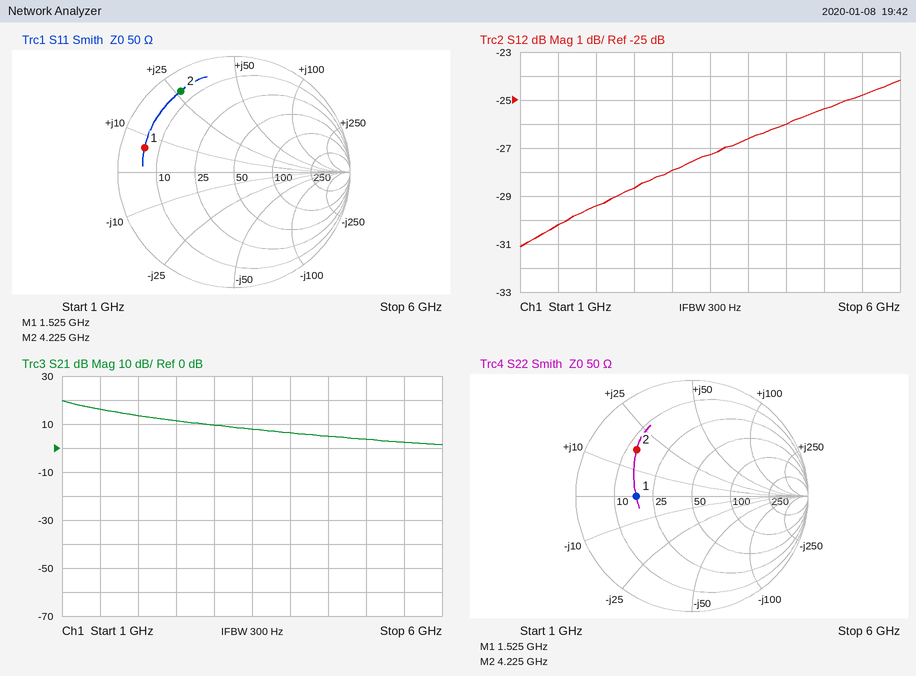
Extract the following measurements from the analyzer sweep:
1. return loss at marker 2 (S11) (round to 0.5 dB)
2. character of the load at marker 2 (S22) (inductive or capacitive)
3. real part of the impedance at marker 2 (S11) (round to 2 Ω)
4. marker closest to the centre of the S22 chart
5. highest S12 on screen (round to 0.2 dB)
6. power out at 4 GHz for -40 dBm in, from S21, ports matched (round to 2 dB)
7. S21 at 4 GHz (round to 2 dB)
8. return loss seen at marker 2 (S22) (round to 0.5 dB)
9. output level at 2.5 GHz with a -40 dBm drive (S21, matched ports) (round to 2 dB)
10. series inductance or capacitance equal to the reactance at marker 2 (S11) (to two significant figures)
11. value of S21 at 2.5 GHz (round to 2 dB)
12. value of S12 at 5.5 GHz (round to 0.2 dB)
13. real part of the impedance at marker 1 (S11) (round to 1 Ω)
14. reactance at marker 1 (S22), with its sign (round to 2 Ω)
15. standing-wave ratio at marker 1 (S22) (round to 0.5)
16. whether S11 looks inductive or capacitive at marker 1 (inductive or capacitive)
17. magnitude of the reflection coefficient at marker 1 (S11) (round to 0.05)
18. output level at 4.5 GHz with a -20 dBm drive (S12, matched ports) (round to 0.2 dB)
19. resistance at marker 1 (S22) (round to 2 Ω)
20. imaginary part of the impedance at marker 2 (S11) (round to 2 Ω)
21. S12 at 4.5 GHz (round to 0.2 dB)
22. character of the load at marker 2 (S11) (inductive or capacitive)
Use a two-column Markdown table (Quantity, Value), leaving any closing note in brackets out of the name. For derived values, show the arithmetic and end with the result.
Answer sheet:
| Quantity | Value |
|---|---|
| return loss at marker 2 (S11) | 1.5 dB |
| character of the load at marker 2 (S22) | inductive |
| real part of the impedance at marker 2 (S11) | 6 Ω |
| marker closest to the centre of the S22 chart | marker 1 |
| highest S12 on screen | -24.2 dB |
| power out at 4 GHz for -40 dBm in, from S21, ports matched | -40 dBm + (6 dB) = -34 dBm |
| S21 at 4 GHz | 6 dB |
| return loss seen at marker 2 (S22) | 4.0 dB |
| output level at 2.5 GHz with a -40 dBm drive (S21, matched ports) | -40 dBm + (12 dB) = -28 dBm |
| series inductance or capacitance equal to the reactance at marker 2 (S11) | L = 26 Ω/(2π × 4.225 GHz) ≈ 1.0 nH |
| value of S21 at 2.5 GHz | 12 dB |
| value of S12 at 5.5 GHz | -24.8 dB |
| real part of the impedance at marker 1 (S11) | 6 Ω |
| reactance at marker 1 (S22), with its sign | 0 Ω |
| standing-wave ratio at marker 1 (S22) | 3.0 |
| whether S11 looks inductive or capacitive at marker 1 | inductive |
| magnitude of the reflection coefficient at marker 1 (S11) | 0.80 |
| output level at 4.5 GHz with a -20 dBm drive (S12, matched ports) | -20 dBm + (-26.0 dB) = -46.0 dBm |
| resistance at marker 1 (S22) | 18 Ω |
| imaginary part of the impedance at marker 2 (S11) | +26 Ω |
| S12 at 4.5 GHz | -26.0 dB |
| character of the load at marker 2 (S11) | inductive |
